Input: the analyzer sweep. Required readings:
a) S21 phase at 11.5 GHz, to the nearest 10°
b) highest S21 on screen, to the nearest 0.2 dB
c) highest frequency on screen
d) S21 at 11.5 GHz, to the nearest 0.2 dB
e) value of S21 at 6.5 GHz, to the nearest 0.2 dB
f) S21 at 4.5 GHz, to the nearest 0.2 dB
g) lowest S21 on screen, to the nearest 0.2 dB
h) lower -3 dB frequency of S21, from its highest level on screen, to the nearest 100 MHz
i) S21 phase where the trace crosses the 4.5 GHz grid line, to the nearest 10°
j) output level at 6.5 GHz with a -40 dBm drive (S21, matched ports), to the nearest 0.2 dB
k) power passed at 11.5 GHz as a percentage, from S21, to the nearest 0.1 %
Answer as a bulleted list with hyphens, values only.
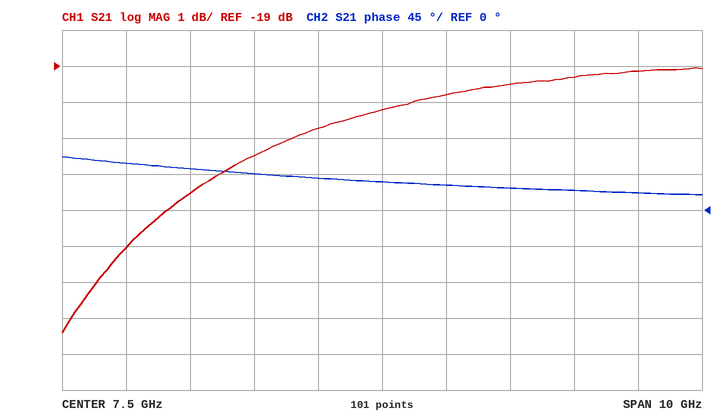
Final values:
- 20°
- -19.0 dB
- 12.5 GHz
- -19.2 dB
- -20.8 dB
- -22.6 dB
- -26.4 dB
- 4.9 GHz
- 50°
- -60.8 dBm
- 1.2 %
